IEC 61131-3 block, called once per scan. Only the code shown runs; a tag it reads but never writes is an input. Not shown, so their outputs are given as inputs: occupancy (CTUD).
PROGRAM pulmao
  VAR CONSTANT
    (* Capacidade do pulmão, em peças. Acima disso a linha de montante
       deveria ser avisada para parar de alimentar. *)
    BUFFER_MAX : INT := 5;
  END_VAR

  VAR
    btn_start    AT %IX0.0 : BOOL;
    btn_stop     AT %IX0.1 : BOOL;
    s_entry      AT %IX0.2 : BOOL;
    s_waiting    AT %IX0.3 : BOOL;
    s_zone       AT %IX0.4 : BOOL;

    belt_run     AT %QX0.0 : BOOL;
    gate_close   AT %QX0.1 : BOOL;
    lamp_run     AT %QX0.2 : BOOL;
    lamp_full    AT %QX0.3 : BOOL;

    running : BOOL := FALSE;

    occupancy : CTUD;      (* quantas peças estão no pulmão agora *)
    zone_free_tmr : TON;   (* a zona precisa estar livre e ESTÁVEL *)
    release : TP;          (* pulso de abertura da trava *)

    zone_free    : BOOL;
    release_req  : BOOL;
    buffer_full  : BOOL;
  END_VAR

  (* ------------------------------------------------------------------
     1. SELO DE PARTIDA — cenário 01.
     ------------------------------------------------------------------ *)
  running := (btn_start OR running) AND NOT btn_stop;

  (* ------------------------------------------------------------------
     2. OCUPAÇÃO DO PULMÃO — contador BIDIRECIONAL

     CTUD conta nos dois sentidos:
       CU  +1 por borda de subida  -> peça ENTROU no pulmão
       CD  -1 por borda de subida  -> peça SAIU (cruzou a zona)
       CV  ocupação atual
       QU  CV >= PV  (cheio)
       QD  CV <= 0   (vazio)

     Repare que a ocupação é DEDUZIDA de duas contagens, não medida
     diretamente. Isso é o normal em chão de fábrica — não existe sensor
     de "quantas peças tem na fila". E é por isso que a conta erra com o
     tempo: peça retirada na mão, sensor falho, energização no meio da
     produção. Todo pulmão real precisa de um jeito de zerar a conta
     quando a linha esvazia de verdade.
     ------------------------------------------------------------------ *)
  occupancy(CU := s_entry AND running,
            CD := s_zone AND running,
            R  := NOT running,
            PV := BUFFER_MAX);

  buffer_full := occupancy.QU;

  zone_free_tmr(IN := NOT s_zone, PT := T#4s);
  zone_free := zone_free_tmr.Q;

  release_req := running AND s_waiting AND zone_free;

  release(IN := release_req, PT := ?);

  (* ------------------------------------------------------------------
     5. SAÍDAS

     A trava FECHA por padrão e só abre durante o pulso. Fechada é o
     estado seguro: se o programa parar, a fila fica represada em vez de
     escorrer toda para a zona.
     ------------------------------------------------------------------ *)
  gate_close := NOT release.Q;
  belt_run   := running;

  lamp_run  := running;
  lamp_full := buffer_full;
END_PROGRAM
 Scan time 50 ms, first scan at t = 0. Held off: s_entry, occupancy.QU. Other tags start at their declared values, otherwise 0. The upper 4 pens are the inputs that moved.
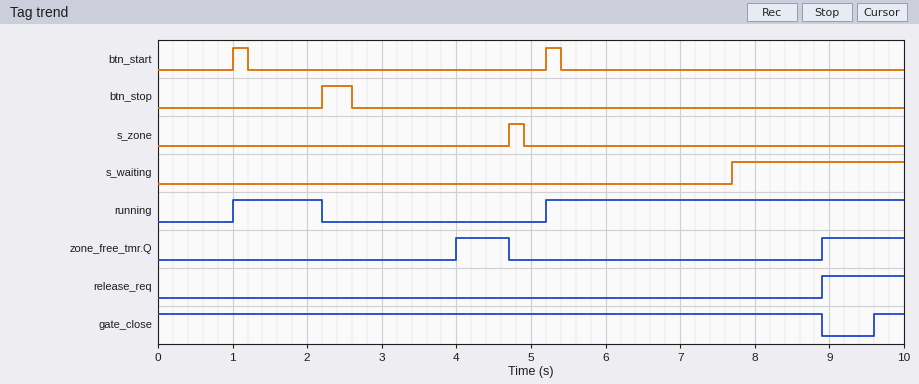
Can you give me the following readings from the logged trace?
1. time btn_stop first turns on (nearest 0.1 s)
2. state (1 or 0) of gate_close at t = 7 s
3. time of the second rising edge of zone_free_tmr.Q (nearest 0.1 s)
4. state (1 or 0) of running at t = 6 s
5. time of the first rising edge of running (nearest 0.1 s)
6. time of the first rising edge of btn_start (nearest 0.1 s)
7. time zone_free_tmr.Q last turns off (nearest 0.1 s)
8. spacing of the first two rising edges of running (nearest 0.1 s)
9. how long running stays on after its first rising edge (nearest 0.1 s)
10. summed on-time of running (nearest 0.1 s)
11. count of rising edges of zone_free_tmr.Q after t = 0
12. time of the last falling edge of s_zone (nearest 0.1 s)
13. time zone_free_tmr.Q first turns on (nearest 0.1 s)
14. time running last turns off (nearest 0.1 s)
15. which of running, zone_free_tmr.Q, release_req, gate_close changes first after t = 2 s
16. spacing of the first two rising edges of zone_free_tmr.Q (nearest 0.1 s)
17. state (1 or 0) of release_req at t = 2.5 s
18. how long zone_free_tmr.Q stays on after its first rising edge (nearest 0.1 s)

2.2 s
1
8.9 s
1
1.0 s
1.0 s
4.7 s
4.2 s
1.2 s
6.0 s
2
4.9 s
4.0 s
2.2 s
running
4.9 s
0
0.7 s
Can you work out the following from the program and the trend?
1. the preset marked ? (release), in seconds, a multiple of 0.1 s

0.7 s
